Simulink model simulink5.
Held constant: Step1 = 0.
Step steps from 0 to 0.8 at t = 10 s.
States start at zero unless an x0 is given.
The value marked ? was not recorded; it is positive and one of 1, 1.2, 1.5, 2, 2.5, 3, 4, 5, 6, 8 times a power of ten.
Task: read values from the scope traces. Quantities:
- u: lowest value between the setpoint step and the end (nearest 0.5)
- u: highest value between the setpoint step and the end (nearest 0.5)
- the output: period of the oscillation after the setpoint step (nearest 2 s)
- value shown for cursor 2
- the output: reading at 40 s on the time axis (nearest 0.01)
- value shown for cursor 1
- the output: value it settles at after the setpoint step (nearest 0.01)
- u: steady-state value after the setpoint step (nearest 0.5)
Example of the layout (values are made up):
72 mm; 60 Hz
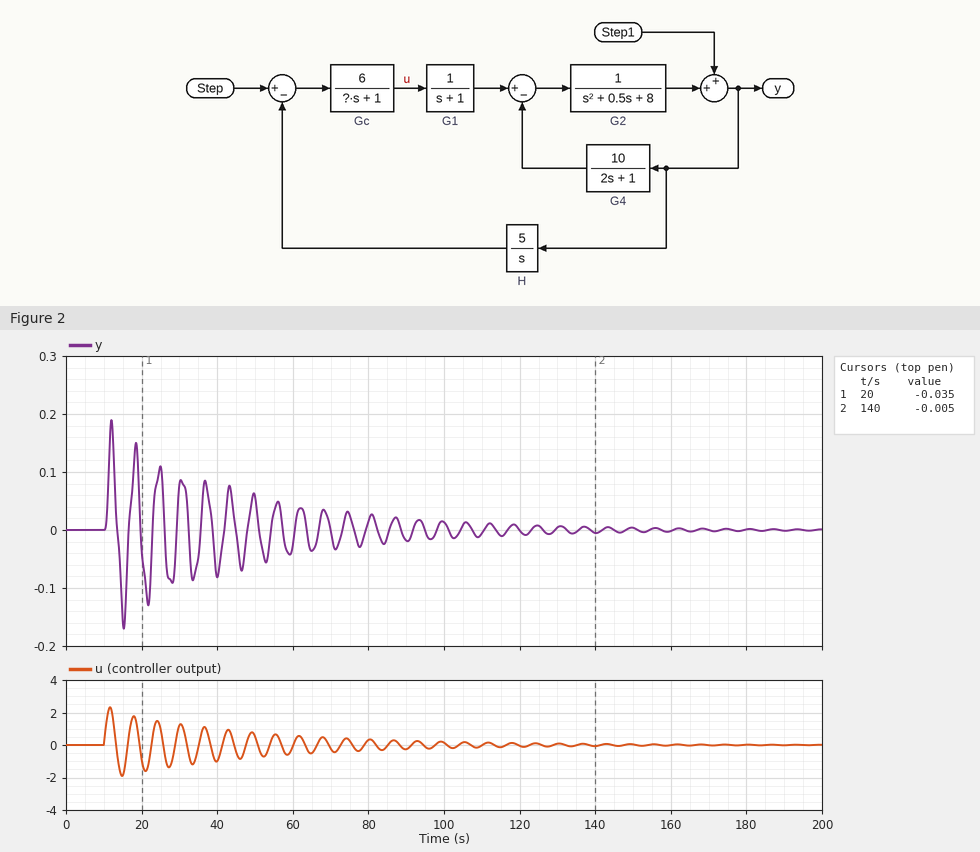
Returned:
-2.0; 2.5; 6 s; -0.005; -0.08; -0.035; 0.00; 0.0
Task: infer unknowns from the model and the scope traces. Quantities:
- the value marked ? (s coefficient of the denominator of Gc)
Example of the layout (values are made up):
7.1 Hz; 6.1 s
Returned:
2
